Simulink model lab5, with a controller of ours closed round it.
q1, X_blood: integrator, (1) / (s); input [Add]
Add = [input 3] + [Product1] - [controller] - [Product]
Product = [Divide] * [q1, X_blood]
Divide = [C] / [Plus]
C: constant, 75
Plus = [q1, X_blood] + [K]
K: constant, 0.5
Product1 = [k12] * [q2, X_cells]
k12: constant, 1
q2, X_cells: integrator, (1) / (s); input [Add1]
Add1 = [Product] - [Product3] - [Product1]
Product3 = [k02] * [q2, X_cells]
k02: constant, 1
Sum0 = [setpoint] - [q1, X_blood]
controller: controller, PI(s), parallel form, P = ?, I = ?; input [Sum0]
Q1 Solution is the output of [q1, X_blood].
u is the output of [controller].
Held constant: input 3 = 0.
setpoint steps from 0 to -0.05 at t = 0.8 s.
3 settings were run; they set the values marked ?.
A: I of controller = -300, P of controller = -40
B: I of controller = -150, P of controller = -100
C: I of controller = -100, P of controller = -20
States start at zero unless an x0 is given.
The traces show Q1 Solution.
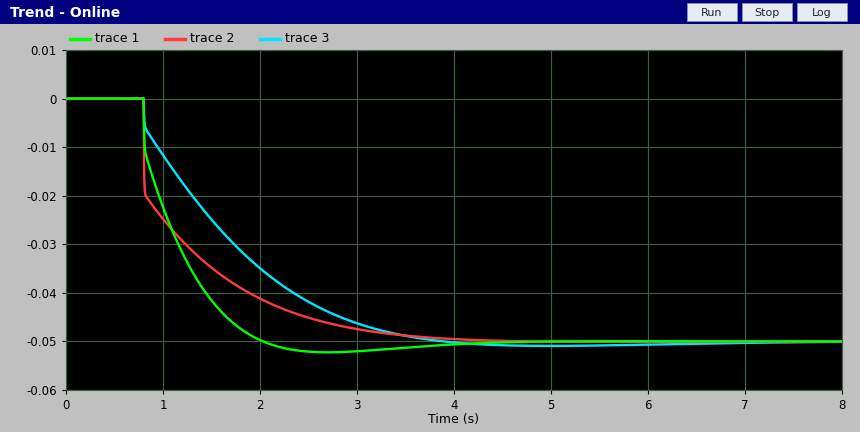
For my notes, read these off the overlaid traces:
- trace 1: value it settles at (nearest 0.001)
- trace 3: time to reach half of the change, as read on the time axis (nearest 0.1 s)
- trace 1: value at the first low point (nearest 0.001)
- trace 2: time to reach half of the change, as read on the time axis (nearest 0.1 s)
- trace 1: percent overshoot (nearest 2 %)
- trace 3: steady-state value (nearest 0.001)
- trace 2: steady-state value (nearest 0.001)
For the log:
-0.050
1.5 s
-0.052
1.0 s
4 %
-0.050
-0.050
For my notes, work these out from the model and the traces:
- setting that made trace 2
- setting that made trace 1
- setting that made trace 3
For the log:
B
A
C
